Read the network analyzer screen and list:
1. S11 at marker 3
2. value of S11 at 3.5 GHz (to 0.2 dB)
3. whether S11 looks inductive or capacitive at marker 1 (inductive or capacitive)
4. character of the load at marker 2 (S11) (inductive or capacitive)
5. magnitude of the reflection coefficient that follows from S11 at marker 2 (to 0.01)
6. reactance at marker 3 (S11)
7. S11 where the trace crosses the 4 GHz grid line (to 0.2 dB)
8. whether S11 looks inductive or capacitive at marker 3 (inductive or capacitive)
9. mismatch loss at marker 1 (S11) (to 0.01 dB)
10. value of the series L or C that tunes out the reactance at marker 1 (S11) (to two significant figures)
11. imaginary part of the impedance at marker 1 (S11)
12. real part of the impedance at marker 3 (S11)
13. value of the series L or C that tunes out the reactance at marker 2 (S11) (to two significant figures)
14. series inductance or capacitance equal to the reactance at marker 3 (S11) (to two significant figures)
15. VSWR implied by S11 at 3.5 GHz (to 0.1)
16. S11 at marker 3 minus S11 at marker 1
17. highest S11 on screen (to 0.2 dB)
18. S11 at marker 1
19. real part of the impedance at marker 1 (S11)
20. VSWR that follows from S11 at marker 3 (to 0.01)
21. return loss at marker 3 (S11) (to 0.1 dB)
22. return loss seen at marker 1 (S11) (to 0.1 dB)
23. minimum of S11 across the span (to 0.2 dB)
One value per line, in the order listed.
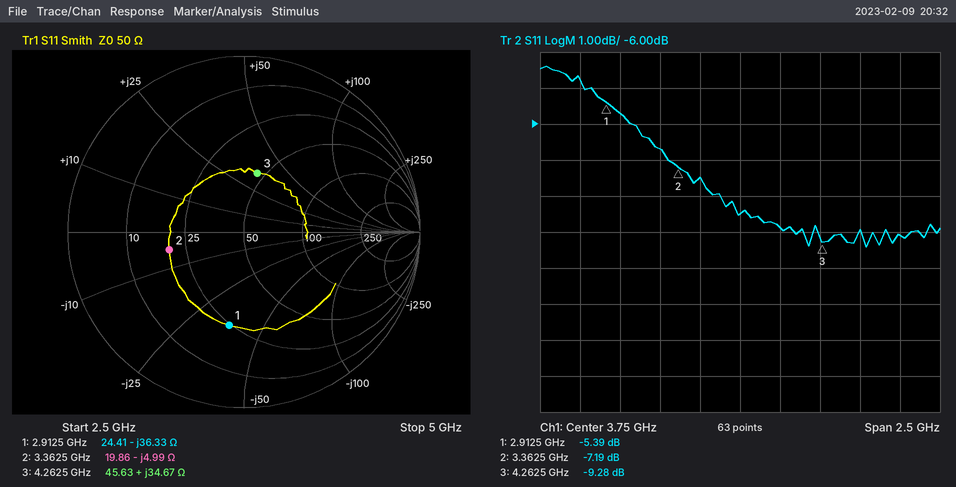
-9.28 dB
-7.4 dB
capacitive
capacitive
0.44
+34.67 Ω
-8.8 dB
inductive
1.48 dB
2.0 nH
-36.33 Ω
45.63 Ω
240 pH
1.3 nH
2.5
-3.89 dB
-4.4 dB
-5.39 dB
24.41 Ω
2.05
9.3 dB
5.4 dB
-9.4 dB
